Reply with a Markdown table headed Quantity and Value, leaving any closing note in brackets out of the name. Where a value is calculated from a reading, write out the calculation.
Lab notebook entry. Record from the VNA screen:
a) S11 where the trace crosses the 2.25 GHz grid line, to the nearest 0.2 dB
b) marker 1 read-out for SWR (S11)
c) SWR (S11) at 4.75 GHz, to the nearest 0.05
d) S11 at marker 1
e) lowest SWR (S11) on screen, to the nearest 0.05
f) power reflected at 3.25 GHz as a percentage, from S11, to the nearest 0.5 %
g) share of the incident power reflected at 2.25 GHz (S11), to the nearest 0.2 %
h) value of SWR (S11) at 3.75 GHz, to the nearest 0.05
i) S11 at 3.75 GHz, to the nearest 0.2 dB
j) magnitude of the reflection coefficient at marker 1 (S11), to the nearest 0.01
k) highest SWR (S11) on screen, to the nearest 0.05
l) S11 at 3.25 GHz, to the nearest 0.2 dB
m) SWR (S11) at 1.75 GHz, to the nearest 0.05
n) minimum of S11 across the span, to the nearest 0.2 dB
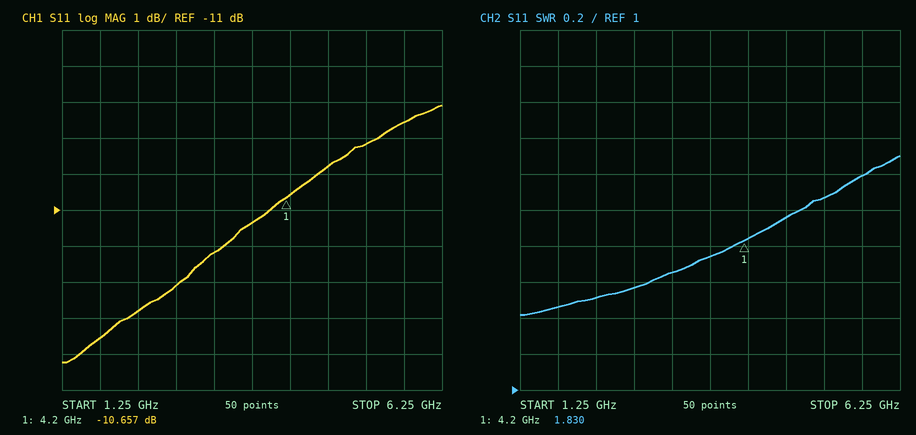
| Quantity | Value |
|---|---|
| S11 where the trace crosses the 2.25 GHz grid line, to the nearest 0.2 dB | -13.8 dB |
| marker 1 read-out for SWR | 1.830 |
| SWR (S11) at 4.75 GHz, to the nearest 0.05 | 1.95 |
| S11 at marker 1 | -10.657 dB |
| lowest SWR (S11) on screen, to the nearest 0.05 | 1.40 |
| power reflected at 3.25 GHz as a percentage, from S11, to the nearest 0.5 % | 10^(-12.2/10) ≈ 6.0 % |
| share of the incident power reflected at 2.25 GHz (S11), to the nearest 0.2 % | 10^(-13.8/10) ≈ 4.2 % |
| value of SWR (S11) at 3.75 GHz, to the nearest 0.05 | 1.75 |
| S11 at 3.75 GHz, to the nearest 0.2 dB | -11.4 dB |
| magnitude of the reflection coefficient at marker 1 (S11), to the nearest 0.01 | 10^(-10.657/20) ≈ 0.29 |
| highest SWR (S11) on screen, to the nearest 0.05 | 2.30 |
| S11 at 3.25 GHz, to the nearest 0.2 dB | -12.2 dB |
| SWR (S11) at 1.75 GHz, to the nearest 0.05 | 1.45 |
| minimum of S11 across the span, to the nearest 0.2 dB | -15.2 dB |
